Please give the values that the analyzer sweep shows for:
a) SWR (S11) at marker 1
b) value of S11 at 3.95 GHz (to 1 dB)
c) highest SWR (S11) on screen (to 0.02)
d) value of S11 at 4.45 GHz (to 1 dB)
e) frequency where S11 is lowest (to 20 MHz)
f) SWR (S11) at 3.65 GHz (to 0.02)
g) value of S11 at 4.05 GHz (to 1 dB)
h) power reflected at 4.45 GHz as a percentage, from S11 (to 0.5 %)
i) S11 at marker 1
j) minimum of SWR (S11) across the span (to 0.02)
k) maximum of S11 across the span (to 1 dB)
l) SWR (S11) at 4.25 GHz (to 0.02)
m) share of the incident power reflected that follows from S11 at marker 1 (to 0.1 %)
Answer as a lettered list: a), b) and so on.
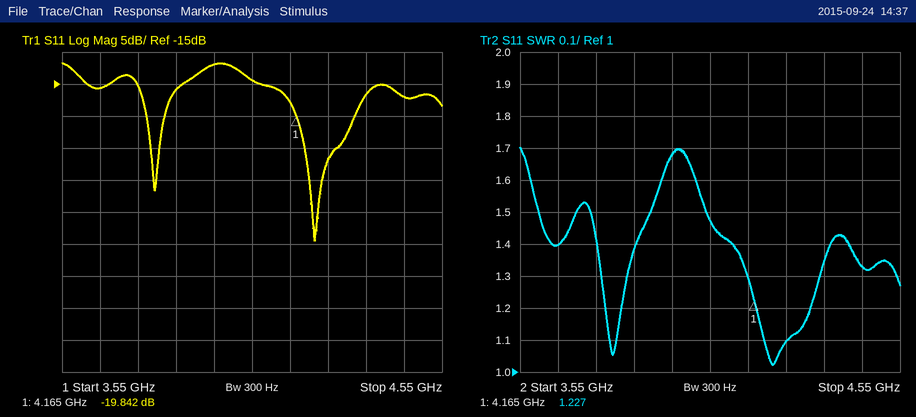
a) 1.227
b) -12 dB
c) 1.70
d) -17 dB
e) 4.22 GHz
f) 1.40
g) -14 dB
h) 2.0 %
i) -19.842 dB
j) 1.02
k) -12 dB
l) 1.10
m) 1.0 %
